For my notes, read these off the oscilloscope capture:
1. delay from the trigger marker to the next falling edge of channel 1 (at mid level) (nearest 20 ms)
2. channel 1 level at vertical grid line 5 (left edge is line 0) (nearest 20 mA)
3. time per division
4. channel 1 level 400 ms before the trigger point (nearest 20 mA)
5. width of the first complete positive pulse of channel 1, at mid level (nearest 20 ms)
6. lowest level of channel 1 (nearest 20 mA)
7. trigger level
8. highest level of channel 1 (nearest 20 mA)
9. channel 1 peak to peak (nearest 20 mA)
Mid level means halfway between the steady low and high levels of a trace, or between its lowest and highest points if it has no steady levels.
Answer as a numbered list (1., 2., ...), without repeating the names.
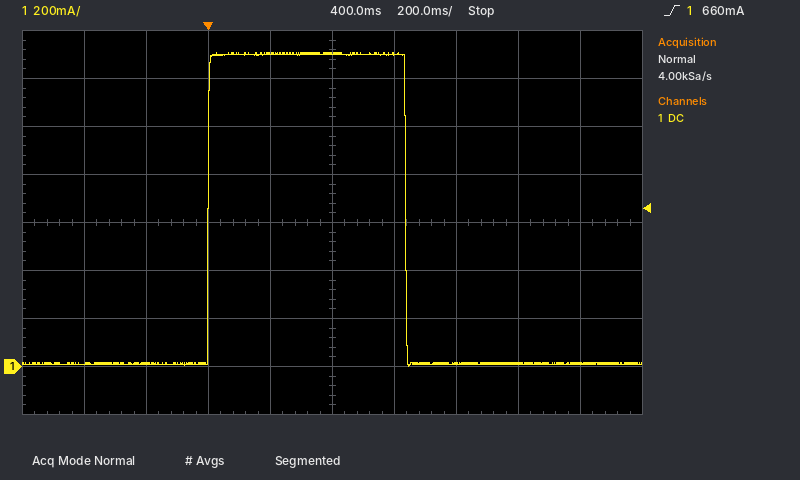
1. 640 ms
2. 1.30 A
3. 200 ms
4. 20 mA
5. 640 ms
6. 0 mA
7. 660 mA
8. 1.30 A
9. 1.30 A
